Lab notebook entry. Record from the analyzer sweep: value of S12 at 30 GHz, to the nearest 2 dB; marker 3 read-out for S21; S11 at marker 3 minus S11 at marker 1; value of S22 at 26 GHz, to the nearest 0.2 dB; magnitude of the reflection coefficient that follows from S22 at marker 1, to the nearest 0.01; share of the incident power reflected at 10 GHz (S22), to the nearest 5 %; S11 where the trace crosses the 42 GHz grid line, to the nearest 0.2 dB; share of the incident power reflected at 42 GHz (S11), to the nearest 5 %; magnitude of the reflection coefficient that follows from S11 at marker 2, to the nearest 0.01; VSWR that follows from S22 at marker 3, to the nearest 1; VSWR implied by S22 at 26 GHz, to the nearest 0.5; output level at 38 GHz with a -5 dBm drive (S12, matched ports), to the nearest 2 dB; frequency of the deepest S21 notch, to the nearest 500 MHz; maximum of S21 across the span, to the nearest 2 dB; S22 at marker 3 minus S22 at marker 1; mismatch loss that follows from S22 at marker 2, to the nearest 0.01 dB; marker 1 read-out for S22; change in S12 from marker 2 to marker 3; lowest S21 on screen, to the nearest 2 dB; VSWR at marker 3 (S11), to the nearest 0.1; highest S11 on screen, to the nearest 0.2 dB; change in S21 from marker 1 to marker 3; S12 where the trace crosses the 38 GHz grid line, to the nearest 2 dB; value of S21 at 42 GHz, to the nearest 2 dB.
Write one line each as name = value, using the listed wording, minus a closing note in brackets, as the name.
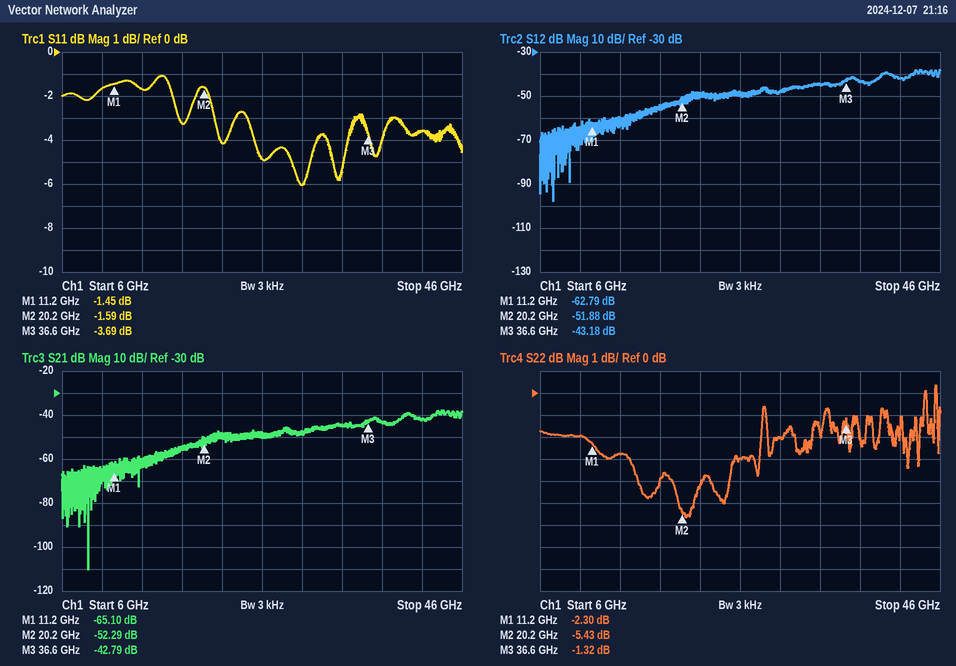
value of S12 at 30 GHz, to the nearest 2 dB = -48 dB
marker 3 read-out for S21 = -42.79 dB
S11 at marker 3 minus S11 at marker 1 = -2.24 dB
value of S22 at 26 GHz, to the nearest 0.2 dB = -3.0 dB
magnitude of the reflection coefficient that follows from S22 at marker 1, to the nearest 0.01 = 0.77
share of the incident power reflected at 10 GHz (S22), to the nearest 5 % = 65 %
S11 where the trace crosses the 42 GHz grid line, to the nearest 0.2 dB = -3.6 dB
share of the incident power reflected at 42 GHz (S11), to the nearest 5 % = 45 %
magnitude of the reflection coefficient that follows from S11 at marker 2, to the nearest 0.01 = 0.83
VSWR that follows from S22 at marker 3, to the nearest 1 = 13
VSWR implied by S22 at 26 GHz, to the nearest 0.5 = 6.0
output level at 38 GHz with a -5 dBm drive (S12, matched ports), to the nearest 2 dB = -48 dBm
frequency of the deepest S21 notch, to the nearest 500 MHz = 8.5 GHz
maximum of S21 across the span, to the nearest 2 dB = -38 dB
S22 at marker 3 minus S22 at marker 1 = 0.98 dB
mismatch loss that follows from S22 at marker 2, to the nearest 0.01 dB = 1.47 dB
marker 1 read-out for S22 = -2.30 dB
change in S12 from marker 2 to marker 3 = 8.70 dB
lowest S21 on screen, to the nearest 2 dB = -110 dB
VSWR at marker 3 (S11), to the nearest 0.1 = 4.8
highest S11 on screen, to the nearest 0.2 dB = -1.0 dB
change in S21 from marker 1 to marker 3 = 22.31 dB
S12 where the trace crosses the 38 GHz grid line, to the nearest 2 dB = -44 dB
value of S21 at 42 GHz, to the nearest 2 dB = -42 dB
